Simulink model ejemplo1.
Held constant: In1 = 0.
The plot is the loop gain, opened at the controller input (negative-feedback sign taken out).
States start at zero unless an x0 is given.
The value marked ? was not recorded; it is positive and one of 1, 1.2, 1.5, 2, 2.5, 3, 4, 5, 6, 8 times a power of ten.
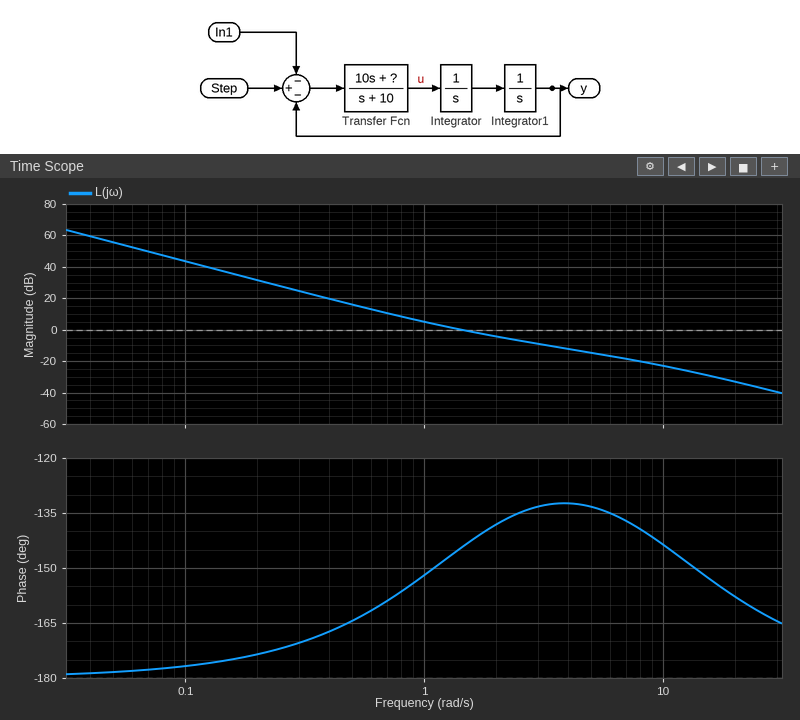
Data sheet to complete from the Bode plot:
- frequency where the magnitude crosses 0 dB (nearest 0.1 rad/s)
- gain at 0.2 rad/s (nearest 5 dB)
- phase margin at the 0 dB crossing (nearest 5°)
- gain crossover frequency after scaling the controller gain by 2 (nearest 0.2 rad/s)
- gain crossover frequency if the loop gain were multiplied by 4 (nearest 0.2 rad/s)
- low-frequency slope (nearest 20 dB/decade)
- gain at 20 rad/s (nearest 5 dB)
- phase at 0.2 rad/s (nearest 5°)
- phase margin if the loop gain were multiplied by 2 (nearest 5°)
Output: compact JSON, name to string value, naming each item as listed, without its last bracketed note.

{"frequency where the magnitude crosses 0 dB": "1.4 rad/s", "gain at 0.2 rad/s": "30 dB", "phase margin at the 0 dB crossing": "35°", "gain crossover frequency after scaling the controller gain by 2": "2.4 rad/s", "gain crossover frequency if the loop gain were multiplied by 4": "4.0 rad/s", "low-frequency slope": "-40 dB/decade", "gain at 20 rad/s": "-35 dB", "phase at 0.2 rad/s": "-175°", "phase margin if the loop gain were multiplied by 2": "45°"}
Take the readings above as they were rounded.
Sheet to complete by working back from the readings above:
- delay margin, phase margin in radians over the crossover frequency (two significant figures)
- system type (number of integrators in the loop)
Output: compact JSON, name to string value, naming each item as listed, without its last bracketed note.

{"delay margin, phase margin in radians over the crossover frequency": "0.44 s", "system type": "2"}
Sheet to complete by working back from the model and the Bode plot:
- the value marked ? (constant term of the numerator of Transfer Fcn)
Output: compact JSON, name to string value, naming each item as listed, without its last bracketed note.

{"the value marked ?": "15"}
